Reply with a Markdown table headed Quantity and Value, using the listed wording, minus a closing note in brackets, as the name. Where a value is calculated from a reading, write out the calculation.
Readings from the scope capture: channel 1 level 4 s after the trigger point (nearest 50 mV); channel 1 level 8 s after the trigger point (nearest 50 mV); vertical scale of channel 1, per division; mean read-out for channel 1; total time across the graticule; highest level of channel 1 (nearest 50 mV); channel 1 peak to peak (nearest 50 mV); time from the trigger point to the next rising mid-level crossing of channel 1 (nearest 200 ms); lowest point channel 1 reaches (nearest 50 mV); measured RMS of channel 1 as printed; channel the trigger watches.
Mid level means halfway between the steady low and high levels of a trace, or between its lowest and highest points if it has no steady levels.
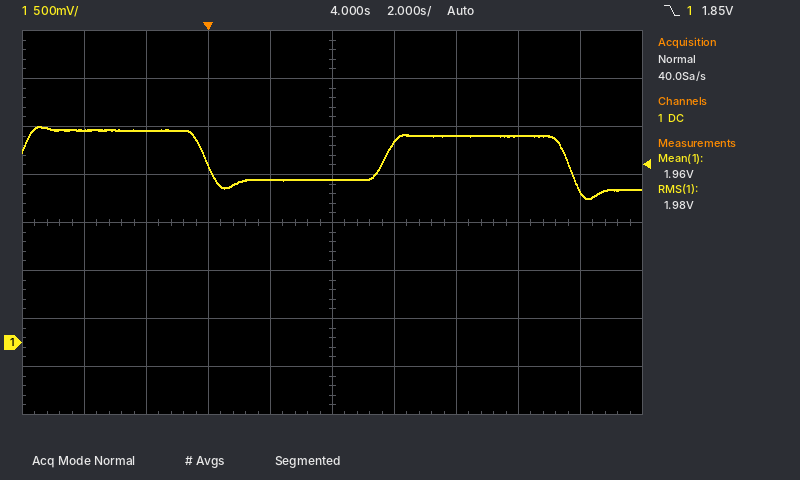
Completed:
| Quantity | Value |
|---|---|
| channel 1 level 4 s after the trigger point | 1.70 V |
| channel 1 level 8 s after the trigger point | 2.15 V |
| vertical scale of channel 1, per division | 500 mV |
| mean read-out for channel 1 | 1.96 V |
| total time across the graticule | 20 s |
| highest level of channel 1 | 2.25 V |
| channel 1 peak to peak | 2.25 V − (1.50 V) = 750 mV |
| time from the trigger point to the next rising mid-level crossing of channel 1 | 5.6 s |
| lowest point channel 1 reaches | 1.50 V |
| measured RMS of channel 1 as printed | 1.98 V |
| channel the trigger watches | channel 1 |
